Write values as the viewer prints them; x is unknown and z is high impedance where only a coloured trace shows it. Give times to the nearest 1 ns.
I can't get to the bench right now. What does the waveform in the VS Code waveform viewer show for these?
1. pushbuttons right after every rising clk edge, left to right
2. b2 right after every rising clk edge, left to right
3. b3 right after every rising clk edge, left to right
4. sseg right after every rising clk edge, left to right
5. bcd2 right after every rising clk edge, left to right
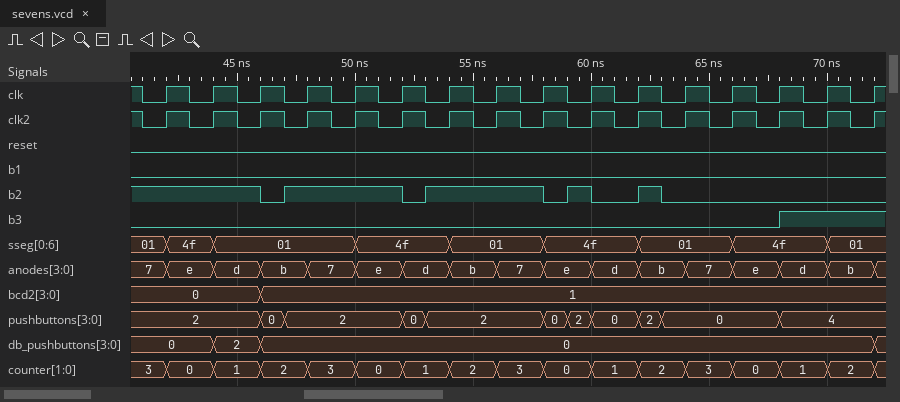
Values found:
2, 2, 0, 2, 2, 0, 2, 2, 0, 0, 2, 0, 0, 4, 4, 4
1 1 0 1 1 0 1 1 0 0 1 0 0 0 0 0
0 0 0 0 0 0 0 0 0 0 0 0 0 1 1 1
4f, 01, 01, 01, 4f, 4f, 01, 01, 4f, 4f, 01, 01, 4f, 4f, 01, 01
0, 0, 1, 1, 1, 1, 1, 1, 1, 1, 1, 1, 1, 1, 1, 1
